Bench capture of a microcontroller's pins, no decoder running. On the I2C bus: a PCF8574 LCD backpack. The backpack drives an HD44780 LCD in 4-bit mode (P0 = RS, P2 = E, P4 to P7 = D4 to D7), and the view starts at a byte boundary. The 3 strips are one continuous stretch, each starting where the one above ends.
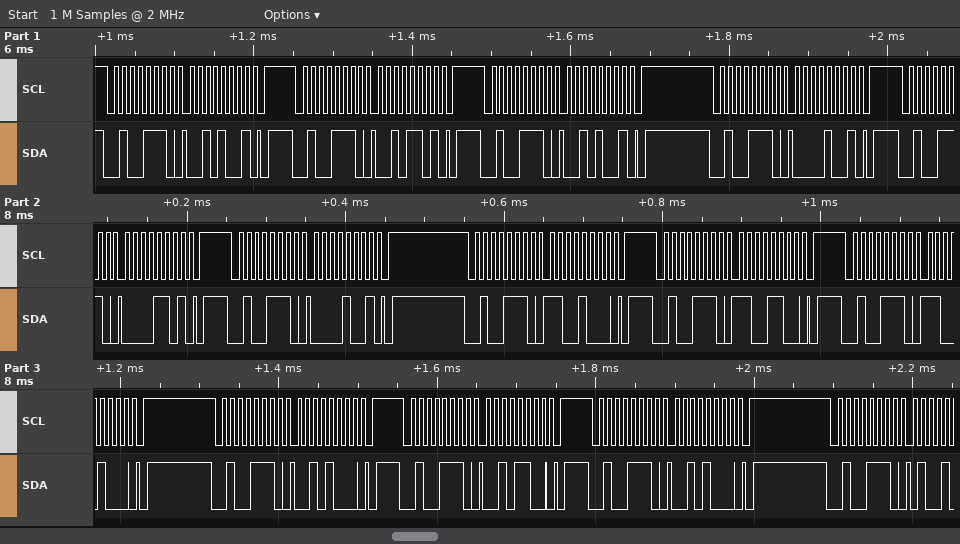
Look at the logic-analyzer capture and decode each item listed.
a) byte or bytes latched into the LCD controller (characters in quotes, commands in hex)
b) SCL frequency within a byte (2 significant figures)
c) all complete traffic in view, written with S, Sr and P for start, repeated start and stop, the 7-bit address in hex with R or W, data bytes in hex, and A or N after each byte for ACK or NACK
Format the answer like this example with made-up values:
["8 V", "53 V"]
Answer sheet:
["' ' 0xC2", "100 kHz", "S 27W A 29 A P S 27W A 2D A P S 27W A 29 A P S 27W A 09 A P S 27W A 0D A P S 27W A 09 A P S 27W A C8 A P S 27W A CC A P S 27W A C8 A P S 27W A 28 A P S 27W A 2C A P S 27W A 28 A P S 27W A"]
